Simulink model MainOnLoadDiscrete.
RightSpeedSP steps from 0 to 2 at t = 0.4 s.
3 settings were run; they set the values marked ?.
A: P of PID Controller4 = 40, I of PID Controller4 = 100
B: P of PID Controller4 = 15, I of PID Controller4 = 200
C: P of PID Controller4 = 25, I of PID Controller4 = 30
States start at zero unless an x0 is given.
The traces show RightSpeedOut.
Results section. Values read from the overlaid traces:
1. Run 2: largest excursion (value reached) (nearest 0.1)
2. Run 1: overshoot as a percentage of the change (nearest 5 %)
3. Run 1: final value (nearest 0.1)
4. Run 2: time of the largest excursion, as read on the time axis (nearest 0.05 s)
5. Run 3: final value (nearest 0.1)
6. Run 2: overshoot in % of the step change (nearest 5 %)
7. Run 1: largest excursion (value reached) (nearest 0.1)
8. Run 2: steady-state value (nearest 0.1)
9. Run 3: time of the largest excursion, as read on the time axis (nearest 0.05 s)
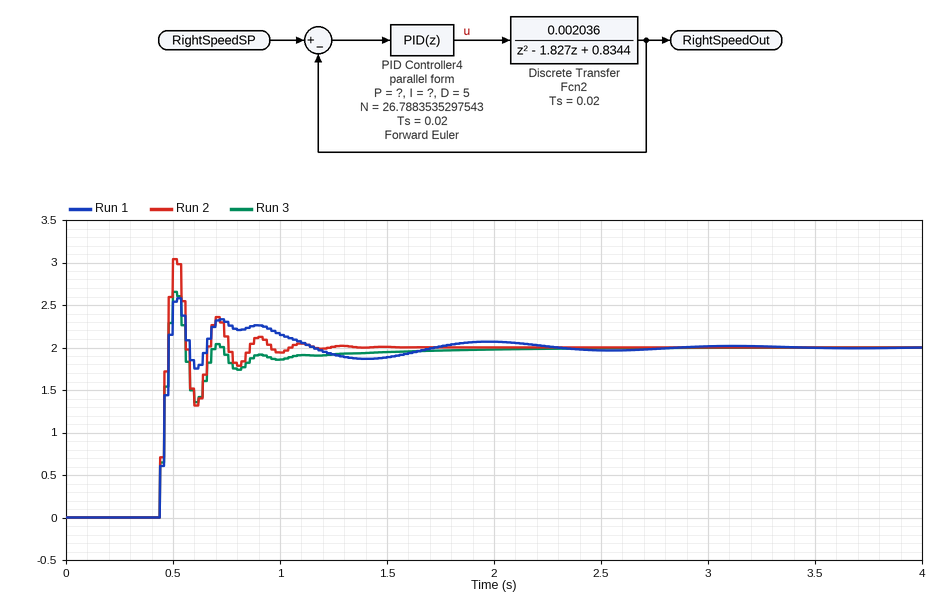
3.0
30 %
2.0
0.50 s
2.0
50 %
2.6
2.0
0.50 s
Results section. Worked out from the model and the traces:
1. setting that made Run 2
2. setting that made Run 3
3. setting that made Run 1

A
C
B
